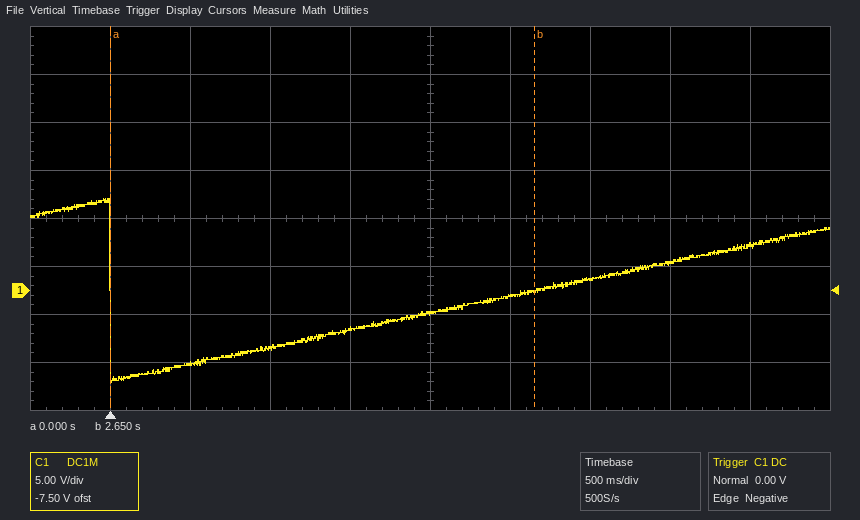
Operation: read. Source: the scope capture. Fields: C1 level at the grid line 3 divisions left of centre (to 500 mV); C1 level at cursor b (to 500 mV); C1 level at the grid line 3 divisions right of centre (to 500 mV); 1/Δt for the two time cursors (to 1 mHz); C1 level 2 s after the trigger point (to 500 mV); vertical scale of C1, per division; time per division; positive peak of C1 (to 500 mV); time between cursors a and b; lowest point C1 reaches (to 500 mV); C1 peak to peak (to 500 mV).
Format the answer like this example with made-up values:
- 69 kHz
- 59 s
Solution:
- -7.5 V
- 0.0 V
- 3.0 V
- 377 mHz
- -2.5 V
- 5 V
- 500 ms
- 9.5 V
- 2.65 s
- -9.5 V
- 19.0 V
